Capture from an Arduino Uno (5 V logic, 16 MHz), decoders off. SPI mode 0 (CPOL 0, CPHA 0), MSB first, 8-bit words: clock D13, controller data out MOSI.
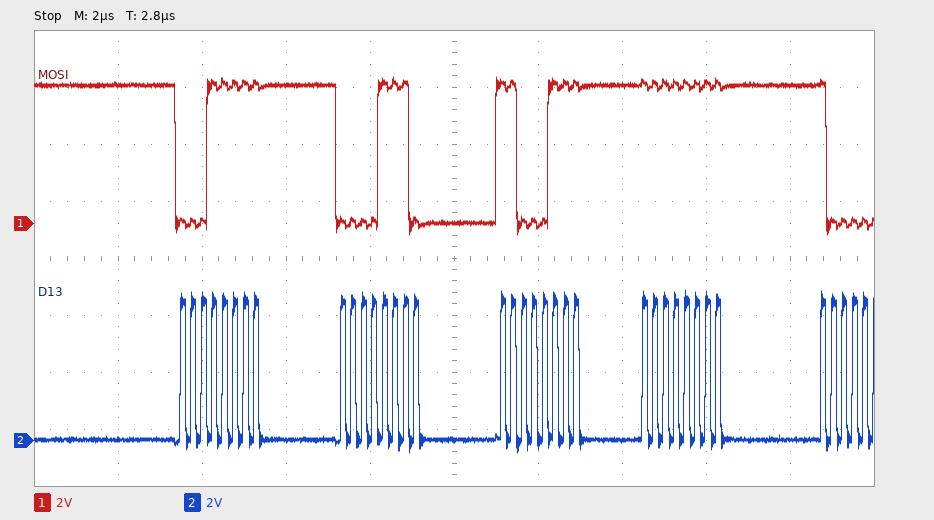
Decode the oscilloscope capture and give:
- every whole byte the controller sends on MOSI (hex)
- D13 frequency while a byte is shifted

1F 0E C7 FF
4 MHz
